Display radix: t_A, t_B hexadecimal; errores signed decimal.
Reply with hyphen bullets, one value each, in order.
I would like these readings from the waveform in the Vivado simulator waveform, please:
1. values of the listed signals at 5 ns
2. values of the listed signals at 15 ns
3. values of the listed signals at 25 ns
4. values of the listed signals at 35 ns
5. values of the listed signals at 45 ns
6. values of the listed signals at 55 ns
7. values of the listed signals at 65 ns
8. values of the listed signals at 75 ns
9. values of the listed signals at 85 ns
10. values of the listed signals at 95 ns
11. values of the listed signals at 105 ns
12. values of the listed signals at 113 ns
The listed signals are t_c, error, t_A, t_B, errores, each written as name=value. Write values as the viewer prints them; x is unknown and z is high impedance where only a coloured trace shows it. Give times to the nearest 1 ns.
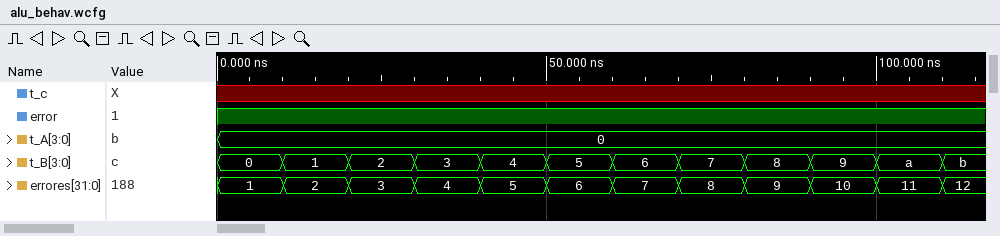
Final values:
- t_c=x, error=1, t_A=0, t_B=0, errores=1
- t_c=x, error=1, t_A=0, t_B=1, errores=2
- t_c=x, error=1, t_A=0, t_B=2, errores=3
- t_c=x, error=1, t_A=0, t_B=3, errores=4
- t_c=x, error=1, t_A=0, t_B=4, errores=5
- t_c=x, error=1, t_A=0, t_B=5, errores=6
- t_c=x, error=1, t_A=0, t_B=6, errores=7
- t_c=x, error=1, t_A=0, t_B=7, errores=8
- t_c=x, error=1, t_A=0, t_B=8, errores=9
- t_c=x, error=1, t_A=0, t_B=9, errores=10
- t_c=x, error=1, t_A=0, t_B=a, errores=11
- t_c=x, error=1, t_A=0, t_B=b, errores=12
